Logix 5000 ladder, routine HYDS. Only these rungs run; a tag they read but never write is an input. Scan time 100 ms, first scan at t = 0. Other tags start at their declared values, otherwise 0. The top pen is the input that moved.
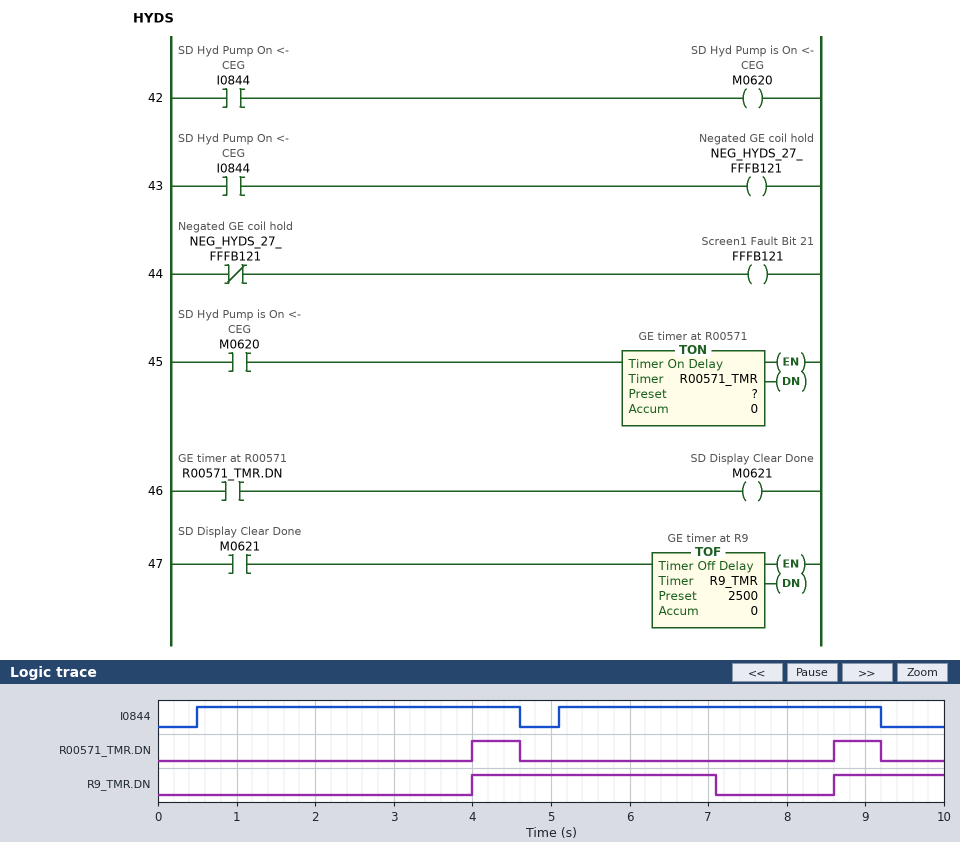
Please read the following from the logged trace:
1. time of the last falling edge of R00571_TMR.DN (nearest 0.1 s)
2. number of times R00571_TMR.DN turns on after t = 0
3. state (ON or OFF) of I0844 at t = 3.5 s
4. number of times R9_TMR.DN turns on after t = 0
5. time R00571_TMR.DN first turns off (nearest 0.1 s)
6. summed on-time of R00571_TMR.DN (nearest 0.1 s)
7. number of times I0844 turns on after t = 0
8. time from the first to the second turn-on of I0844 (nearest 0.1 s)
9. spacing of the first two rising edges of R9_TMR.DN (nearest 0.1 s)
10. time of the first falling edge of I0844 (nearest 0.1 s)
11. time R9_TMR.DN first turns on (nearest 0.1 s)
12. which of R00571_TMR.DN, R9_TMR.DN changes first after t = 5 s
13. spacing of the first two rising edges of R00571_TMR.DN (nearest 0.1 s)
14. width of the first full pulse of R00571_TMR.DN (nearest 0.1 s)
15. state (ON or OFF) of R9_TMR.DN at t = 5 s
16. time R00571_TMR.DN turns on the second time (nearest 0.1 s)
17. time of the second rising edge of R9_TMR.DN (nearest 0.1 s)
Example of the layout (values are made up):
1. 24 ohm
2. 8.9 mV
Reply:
1. 9.2 s
2. 2
3. ON
4. 2
5. 4.6 s
6. 1.2 s
7. 2
8. 4.6 s
9. 4.6 s
10. 4.6 s
11. 4.0 s
12. R9_TMR.DN
13. 4.6 s
14. 0.6 s
15. ON
16. 8.6 s
17. 8.6 s
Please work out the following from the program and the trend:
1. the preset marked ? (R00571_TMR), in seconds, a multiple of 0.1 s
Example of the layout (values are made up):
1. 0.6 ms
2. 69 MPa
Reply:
1. 3.5 s
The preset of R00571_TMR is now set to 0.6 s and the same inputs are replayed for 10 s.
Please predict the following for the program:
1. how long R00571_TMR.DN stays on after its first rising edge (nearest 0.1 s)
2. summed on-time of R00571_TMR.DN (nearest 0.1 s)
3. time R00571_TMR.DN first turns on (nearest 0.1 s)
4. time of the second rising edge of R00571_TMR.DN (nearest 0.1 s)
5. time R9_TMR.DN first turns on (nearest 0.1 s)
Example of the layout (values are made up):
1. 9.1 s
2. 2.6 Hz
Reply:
1. 3.5 s
2. 7.0 s
3. 1.1 s
4. 5.7 s
5. 1.1 s
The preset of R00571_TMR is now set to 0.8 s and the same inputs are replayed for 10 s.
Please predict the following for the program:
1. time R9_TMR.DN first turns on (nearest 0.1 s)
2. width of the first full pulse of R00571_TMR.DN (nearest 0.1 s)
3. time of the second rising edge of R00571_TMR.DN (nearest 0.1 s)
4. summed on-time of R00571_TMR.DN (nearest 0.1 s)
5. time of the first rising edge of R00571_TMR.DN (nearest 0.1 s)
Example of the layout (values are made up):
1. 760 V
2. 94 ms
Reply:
1. 1.3 s
2. 3.3 s
3. 5.9 s
4. 6.6 s
5. 1.3 s
